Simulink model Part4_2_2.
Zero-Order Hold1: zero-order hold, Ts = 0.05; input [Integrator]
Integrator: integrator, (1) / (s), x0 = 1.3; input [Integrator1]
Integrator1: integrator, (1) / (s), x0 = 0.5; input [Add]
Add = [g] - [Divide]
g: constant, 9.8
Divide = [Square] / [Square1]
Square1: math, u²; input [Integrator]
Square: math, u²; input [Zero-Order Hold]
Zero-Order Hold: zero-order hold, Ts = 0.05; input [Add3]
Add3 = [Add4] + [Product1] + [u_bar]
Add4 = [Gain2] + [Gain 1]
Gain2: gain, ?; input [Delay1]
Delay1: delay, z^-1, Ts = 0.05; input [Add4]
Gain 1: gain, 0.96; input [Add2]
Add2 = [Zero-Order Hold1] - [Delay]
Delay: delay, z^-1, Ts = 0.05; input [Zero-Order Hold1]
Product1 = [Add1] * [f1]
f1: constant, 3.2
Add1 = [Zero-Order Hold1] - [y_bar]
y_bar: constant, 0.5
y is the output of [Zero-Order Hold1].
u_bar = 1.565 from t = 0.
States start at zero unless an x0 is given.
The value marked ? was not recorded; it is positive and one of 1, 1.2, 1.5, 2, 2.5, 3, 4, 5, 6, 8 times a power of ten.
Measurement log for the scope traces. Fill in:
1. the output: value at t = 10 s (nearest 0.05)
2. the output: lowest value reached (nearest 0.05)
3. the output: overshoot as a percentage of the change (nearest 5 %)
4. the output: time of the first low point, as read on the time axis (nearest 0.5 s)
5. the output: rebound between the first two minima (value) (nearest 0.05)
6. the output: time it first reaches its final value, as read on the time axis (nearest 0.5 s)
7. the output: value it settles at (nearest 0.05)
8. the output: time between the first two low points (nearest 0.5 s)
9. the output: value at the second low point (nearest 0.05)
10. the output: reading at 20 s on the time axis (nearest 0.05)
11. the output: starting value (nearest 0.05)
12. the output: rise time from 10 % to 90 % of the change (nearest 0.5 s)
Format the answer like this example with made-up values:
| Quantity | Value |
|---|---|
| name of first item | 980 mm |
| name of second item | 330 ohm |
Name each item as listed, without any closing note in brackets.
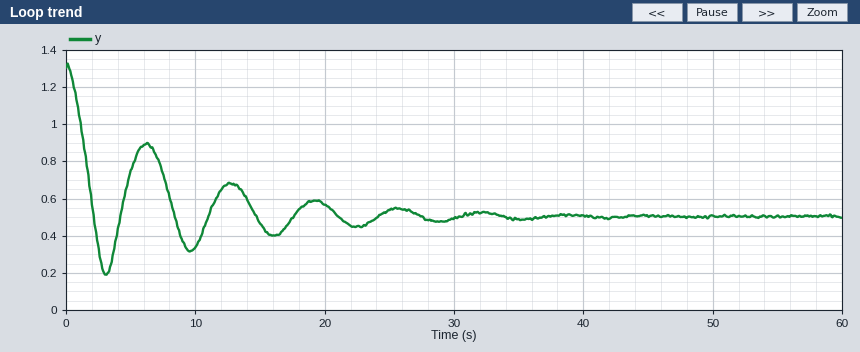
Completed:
| Quantity | Value |
|---|---|
| the output: value at t = 10 s | 0.35 |
| the output: lowest value reached | 0.20 |
| the output: overshoot as a percentage of the change | 40 % |
| the output: time of the first low point, as read on the time axis | 3.0 s |
| the output: rebound between the first two minima (value) | 0.90 |
| the output: time it first reaches its final value, as read on the time axis | 2.0 s |
| the output: value it settles at | 0.50 |
| the output: time between the first two low points | 6.5 s |
| the output: value at the second low point | 0.30 |
| the output: reading at 20 s on the time axis | 0.55 |
| the output: starting value | 1.30 |
| the output: rise time from 10 % to 90 % of the change | 1.5 s |
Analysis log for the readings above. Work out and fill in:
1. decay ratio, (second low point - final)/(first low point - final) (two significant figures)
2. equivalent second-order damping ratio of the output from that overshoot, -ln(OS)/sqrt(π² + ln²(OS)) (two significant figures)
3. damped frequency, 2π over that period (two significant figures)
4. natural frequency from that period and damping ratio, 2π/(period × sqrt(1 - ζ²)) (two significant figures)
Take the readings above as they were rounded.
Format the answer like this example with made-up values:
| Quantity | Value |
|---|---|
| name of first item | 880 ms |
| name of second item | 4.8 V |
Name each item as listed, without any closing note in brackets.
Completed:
| Quantity | Value |
|---|---|
| decay ratio, (second low point - final)/(first low point - final) | 0.67 |
| equivalent second-order damping ratio of the output from that overshoot, -ln(OS)/sqrt(π² + ln²(OS)) | 0.28 |
| damped frequency, 2π over that period | 0.97 rad/s |
| natural frequency from that period and damping ratio, 2π/(period × sqrt(1 - ζ²)) | 1.0 rad/s |
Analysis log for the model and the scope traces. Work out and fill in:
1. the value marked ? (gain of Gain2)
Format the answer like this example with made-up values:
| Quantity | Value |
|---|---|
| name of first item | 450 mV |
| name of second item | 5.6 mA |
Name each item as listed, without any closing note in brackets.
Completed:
| Quantity | Value |
|---|---|
| the value marked ? | 0.5 |
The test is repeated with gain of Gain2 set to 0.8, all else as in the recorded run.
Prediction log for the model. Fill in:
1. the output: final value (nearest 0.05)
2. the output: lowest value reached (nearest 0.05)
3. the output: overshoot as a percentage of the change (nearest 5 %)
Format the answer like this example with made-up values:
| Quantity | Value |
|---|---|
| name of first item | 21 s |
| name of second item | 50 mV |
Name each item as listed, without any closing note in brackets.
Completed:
| Quantity | Value |
|---|---|
| the output: final value | 0.50 |
| the output: lowest value reached | 0.35 |
| the output: overshoot as a percentage of the change | 20 % |
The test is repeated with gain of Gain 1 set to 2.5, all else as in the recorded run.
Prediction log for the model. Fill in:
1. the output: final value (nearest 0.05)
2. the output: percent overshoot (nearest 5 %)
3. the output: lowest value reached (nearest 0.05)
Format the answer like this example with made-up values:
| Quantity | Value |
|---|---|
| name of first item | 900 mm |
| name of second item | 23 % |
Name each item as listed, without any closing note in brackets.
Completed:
| Quantity | Value |
|---|---|
| the output: final value | 0.50 |
| the output: percent overshoot | 20 % |
| the output: lowest value reached | 0.35 |
